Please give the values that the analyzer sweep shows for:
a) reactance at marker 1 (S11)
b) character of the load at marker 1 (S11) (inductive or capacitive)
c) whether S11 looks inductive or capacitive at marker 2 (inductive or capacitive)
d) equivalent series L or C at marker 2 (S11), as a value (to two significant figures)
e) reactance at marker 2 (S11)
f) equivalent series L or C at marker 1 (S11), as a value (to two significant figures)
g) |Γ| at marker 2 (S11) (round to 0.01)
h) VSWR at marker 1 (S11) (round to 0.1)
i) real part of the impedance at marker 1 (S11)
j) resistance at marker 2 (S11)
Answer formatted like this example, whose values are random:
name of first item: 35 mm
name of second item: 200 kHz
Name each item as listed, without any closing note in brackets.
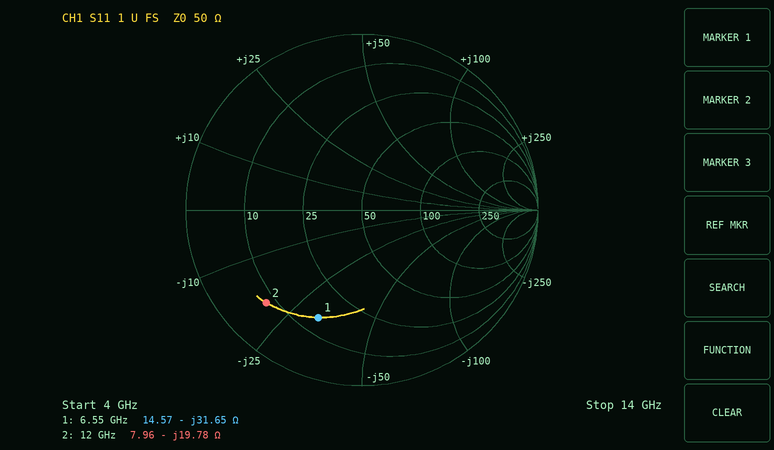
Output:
reactance at marker 1: -31.65 Ω
character of the load at marker 1 (S11): capacitive
whether S11 looks inductive or capacitive at marker 2: capacitive
equivalent series L or C at marker 2 (S11), as a value: 670 fF
reactance at marker 2: -19.78 Ω
equivalent series L or C at marker 1 (S11), as a value: 770 fF
|Γ| at marker 2 (S11): 0.76
VSWR at marker 1 (S11): 4.9
real part of the impedance at marker 1: 14.57 Ω
resistance at marker 2: 7.96 Ω
